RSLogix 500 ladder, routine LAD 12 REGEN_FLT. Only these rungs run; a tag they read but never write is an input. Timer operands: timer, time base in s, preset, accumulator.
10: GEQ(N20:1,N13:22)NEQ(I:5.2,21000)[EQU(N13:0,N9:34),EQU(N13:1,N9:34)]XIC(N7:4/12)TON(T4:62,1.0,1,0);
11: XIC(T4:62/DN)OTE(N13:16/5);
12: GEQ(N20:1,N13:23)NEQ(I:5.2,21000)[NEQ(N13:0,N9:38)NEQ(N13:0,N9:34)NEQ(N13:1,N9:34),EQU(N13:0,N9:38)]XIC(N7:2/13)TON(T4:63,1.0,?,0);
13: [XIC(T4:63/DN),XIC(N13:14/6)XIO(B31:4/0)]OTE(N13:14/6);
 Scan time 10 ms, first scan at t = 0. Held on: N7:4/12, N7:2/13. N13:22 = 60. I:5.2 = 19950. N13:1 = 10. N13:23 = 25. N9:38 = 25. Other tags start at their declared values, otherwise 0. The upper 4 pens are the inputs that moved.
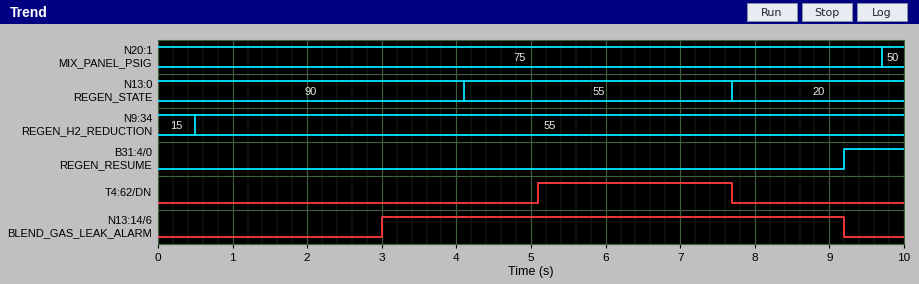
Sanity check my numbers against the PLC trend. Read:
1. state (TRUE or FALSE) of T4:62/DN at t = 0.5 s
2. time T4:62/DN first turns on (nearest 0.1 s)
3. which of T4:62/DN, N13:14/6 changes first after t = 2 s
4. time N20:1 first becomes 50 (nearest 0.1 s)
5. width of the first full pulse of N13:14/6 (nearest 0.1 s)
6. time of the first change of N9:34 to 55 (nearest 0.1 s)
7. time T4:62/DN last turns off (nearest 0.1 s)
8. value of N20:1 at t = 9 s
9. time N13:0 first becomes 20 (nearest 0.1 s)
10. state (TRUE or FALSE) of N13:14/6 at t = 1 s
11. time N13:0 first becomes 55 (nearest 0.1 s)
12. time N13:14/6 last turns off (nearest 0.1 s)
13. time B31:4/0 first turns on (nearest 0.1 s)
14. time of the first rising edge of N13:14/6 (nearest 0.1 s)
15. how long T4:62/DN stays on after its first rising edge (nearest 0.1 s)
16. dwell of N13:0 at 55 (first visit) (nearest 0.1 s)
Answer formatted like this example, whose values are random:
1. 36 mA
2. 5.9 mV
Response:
1. FALSE
2. 5.1 s
3. N13:14/6
4. 9.7 s
5. 6.2 s
6. 0.5 s
7. 7.7 s
8. 75
9. 7.7 s
10. FALSE
11. 4.1 s
12. 9.2 s
13. 9.2 s
14. 3.0 s
15. 2.6 s
16. 3.6 s
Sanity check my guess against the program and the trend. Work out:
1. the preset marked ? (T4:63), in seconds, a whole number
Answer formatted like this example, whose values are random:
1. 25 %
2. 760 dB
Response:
1. 3 s
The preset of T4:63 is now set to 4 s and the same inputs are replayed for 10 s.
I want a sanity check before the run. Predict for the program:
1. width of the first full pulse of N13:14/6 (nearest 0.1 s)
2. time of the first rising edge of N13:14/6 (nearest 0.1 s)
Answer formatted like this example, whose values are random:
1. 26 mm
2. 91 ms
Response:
1. 5.2 s
2. 4.0 s
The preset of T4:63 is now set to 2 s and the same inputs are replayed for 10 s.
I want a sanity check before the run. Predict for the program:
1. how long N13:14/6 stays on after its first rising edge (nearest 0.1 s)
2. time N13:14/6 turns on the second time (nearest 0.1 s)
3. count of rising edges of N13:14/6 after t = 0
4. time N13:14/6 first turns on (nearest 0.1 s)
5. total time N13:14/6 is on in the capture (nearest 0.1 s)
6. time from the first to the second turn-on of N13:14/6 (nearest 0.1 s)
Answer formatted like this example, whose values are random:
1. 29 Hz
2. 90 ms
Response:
1. 7.2 s
2. 9.7 s
3. 2
4. 2.0 s
5. 7.5 s
6. 7.7 s
